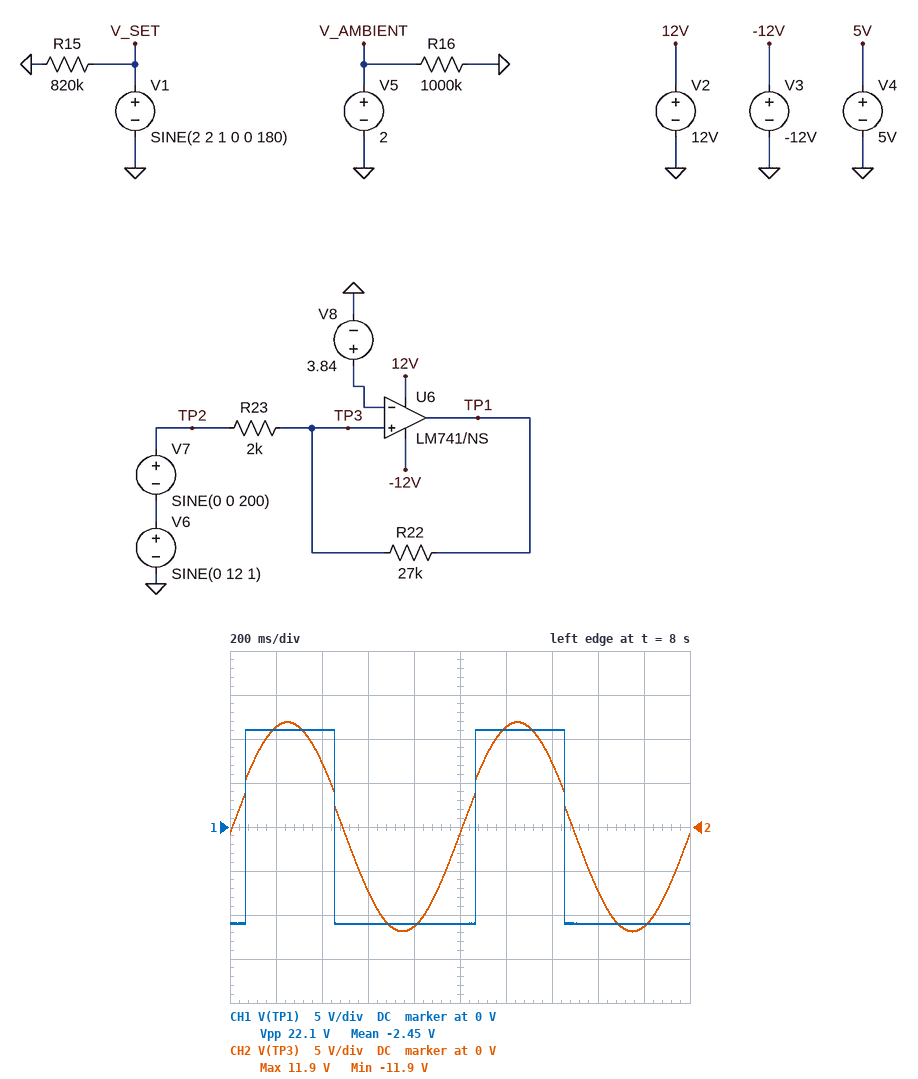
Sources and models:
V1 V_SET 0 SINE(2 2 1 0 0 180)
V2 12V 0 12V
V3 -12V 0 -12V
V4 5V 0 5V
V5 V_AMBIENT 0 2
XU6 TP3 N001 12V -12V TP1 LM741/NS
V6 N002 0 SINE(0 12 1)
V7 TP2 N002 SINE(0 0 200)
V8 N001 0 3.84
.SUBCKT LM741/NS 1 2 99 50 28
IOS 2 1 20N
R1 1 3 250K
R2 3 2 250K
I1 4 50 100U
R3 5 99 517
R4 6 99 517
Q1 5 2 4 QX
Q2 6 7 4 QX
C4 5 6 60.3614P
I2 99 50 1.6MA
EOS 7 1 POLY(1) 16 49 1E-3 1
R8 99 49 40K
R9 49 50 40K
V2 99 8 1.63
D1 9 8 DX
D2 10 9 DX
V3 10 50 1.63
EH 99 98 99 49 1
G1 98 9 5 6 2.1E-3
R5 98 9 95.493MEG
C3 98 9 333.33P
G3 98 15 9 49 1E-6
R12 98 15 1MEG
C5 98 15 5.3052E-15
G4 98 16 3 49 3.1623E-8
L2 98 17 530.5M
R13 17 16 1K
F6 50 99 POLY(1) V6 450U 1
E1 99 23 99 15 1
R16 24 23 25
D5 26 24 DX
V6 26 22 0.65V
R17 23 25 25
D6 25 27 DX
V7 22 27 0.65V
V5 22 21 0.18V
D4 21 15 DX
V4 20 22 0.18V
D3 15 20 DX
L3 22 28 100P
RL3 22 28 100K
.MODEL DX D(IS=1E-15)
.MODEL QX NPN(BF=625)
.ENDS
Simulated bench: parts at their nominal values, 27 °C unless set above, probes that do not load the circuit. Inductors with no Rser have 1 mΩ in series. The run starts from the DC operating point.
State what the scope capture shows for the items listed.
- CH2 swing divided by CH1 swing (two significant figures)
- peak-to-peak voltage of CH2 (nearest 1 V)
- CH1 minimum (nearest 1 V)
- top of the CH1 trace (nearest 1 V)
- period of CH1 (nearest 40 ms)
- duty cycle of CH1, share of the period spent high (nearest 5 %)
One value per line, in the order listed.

1.1
24 V
-11 V
11 V
1.00 s
40 %
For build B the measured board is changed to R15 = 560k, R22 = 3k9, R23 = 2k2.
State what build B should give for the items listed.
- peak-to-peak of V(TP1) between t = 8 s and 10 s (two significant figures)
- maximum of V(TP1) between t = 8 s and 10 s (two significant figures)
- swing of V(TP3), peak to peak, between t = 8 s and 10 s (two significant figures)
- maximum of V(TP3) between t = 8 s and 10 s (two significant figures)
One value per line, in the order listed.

220 mV
-11 V
15 V
3.8 V
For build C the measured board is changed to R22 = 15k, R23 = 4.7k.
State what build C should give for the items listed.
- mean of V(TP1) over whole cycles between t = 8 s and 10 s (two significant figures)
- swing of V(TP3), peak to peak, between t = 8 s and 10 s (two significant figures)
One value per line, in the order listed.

-3.2 V
23 V
